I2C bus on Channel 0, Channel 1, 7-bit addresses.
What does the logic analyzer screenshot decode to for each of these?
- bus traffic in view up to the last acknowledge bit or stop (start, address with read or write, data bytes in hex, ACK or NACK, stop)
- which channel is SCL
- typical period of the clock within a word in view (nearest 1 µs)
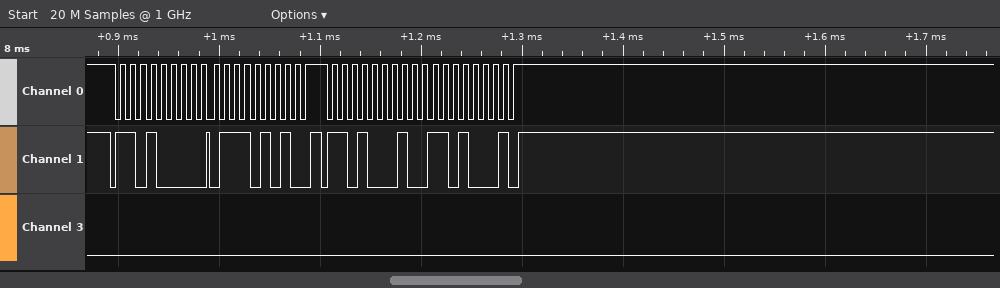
start, address 68 write ACK, 75 ACK, stop, start, address 68 read ACK, 68 NACK, stop
Channel 0
10 µs
